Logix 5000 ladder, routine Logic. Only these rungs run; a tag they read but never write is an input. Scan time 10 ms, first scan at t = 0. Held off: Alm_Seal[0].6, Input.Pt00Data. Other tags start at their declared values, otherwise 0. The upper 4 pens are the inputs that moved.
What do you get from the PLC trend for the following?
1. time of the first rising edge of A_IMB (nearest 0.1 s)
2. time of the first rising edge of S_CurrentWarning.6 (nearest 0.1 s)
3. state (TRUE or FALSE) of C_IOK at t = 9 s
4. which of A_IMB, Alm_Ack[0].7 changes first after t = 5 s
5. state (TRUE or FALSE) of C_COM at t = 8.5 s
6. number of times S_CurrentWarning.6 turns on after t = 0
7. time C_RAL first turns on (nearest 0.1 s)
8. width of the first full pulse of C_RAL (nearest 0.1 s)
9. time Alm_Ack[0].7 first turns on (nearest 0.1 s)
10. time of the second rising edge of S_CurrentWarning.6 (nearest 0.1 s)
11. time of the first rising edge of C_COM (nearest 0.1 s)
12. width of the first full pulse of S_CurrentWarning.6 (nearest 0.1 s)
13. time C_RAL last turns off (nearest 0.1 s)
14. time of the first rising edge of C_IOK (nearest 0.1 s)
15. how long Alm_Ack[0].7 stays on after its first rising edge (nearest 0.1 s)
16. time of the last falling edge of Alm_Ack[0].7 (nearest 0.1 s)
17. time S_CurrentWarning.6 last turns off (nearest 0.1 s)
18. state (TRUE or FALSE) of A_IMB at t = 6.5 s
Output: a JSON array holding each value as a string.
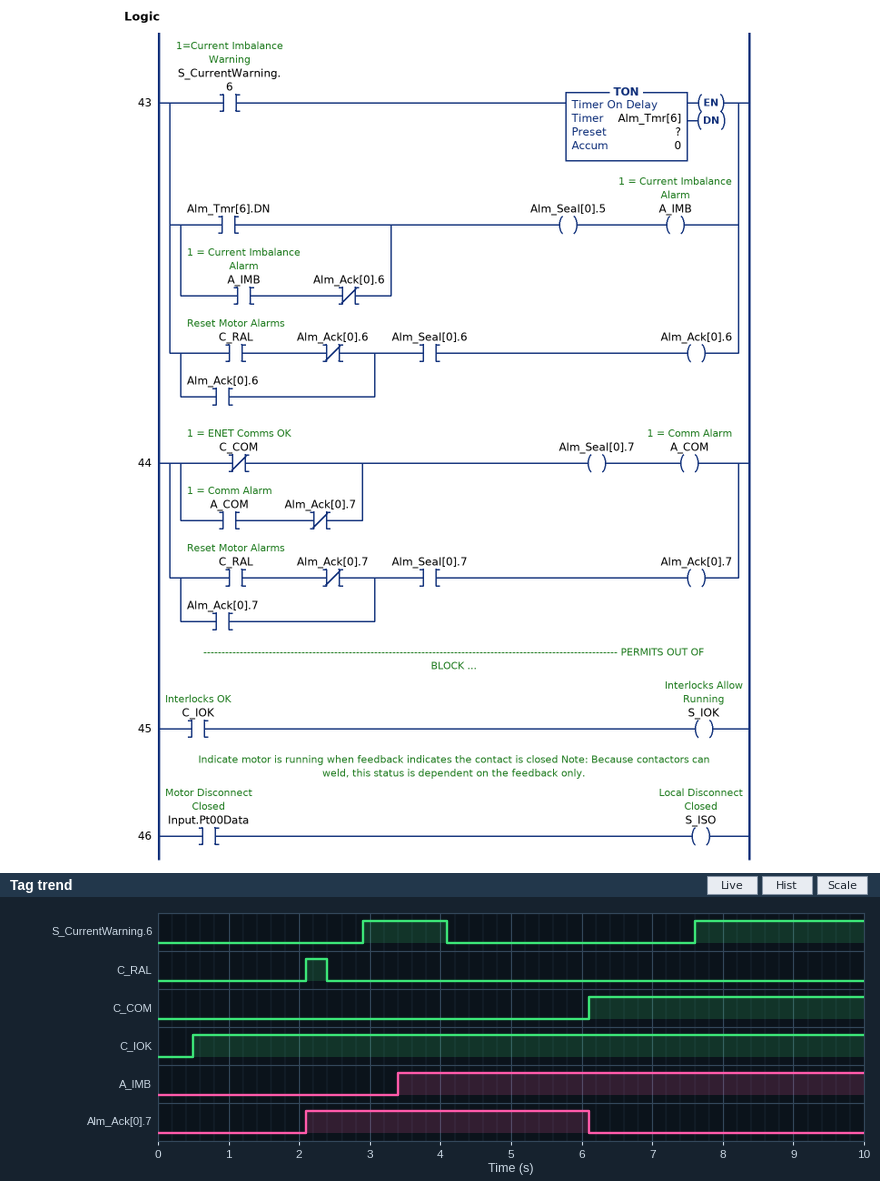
["3.4 s", "2.9 s", "TRUE", "Alm_Ack[0].7", "TRUE", "2", "2.1 s", "0.3 s", "2.1 s", "7.6 s", "6.1 s", "1.2 s", "2.4 s", "0.5 s", "4.0 s", "6.1 s", "4.1 s", "TRUE"]
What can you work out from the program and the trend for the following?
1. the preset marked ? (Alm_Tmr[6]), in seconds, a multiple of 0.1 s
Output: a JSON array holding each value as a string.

["0.5 s"]
